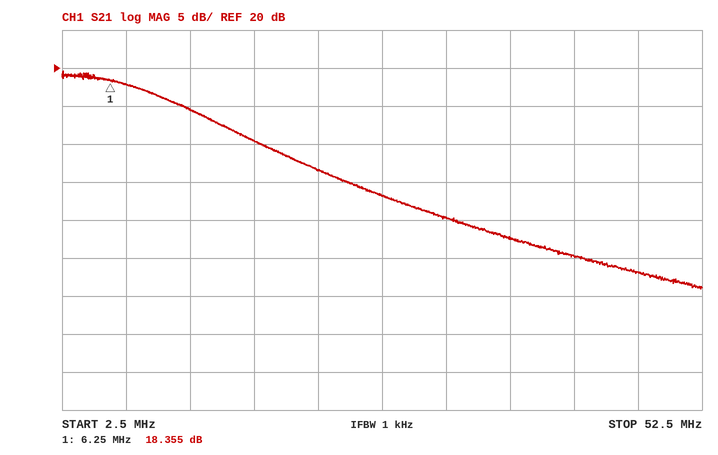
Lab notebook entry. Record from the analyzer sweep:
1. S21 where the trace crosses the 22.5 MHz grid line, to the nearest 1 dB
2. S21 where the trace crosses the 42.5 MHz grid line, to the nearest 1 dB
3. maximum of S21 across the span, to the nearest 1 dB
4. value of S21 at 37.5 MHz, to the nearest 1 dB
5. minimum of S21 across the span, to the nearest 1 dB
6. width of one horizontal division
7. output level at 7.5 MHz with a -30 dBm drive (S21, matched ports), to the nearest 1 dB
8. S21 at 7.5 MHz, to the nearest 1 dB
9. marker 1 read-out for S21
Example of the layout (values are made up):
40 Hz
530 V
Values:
7 dB
-5 dB
20 dB
-2 dB
-9 dB
5 MHz
-12 dBm
18 dB
18.355 dB
